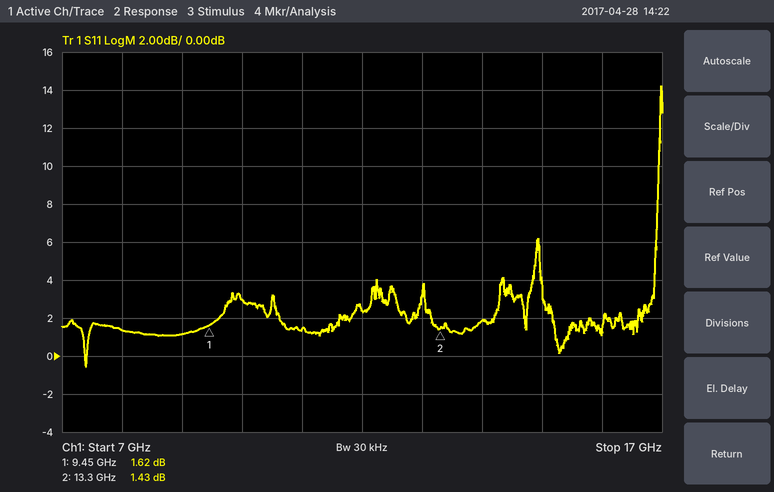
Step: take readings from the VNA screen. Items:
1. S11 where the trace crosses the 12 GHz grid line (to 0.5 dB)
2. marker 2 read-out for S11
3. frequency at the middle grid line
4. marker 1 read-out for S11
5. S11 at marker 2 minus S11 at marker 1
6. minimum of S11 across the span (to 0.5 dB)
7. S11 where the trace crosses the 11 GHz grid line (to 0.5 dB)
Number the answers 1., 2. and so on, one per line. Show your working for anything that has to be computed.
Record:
1. 2.5 dB
2. 1.43 dB
3. 12 GHz
4. 1.62 dB
5. 1.43 − (1.62) = -0.19 dB
6. -0.5 dB
7. 1.5 dB
